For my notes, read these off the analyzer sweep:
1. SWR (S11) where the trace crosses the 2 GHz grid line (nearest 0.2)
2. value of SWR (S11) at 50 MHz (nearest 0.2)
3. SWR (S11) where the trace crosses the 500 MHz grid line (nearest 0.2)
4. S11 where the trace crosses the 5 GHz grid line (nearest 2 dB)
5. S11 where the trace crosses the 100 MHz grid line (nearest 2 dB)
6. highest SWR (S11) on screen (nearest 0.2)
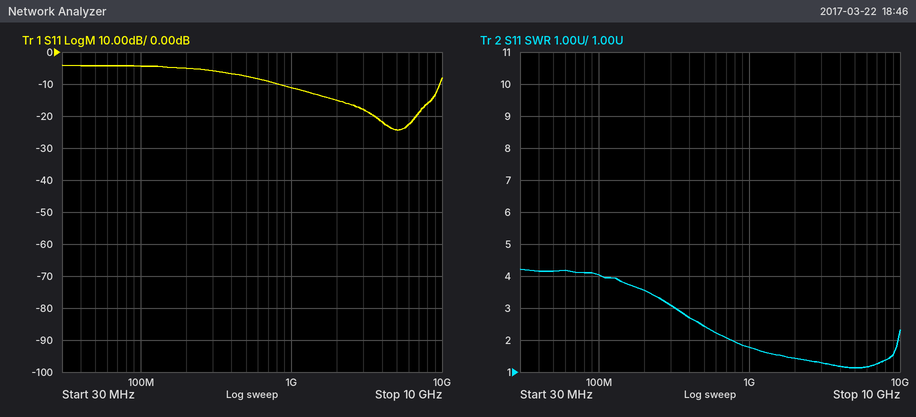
1.4
4.2
2.4
-24 dB
-4 dB
4.2
